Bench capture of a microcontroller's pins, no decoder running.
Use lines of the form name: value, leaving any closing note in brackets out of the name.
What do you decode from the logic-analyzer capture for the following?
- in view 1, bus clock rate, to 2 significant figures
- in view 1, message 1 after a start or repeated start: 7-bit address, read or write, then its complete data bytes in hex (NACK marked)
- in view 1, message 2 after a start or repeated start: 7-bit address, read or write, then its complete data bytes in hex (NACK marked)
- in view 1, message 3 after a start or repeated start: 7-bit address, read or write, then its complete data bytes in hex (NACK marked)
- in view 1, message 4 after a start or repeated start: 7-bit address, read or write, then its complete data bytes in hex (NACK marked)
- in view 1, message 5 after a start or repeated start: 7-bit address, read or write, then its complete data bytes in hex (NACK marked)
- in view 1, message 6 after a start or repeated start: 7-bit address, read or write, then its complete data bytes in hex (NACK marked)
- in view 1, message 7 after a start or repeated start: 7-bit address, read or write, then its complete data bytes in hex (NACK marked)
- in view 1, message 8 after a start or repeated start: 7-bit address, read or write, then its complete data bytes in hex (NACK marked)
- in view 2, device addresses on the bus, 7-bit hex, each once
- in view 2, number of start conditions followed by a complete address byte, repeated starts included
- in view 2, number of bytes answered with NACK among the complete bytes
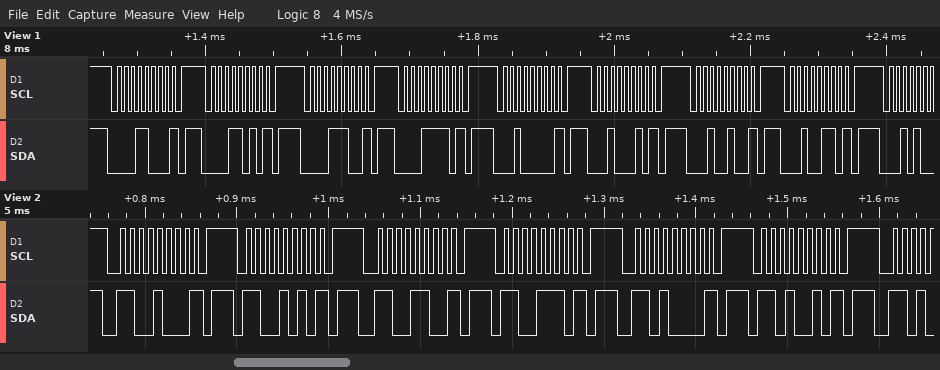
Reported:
in view 1, bus clock rate, to 2 significant figures: 100 kHz
in view 1, message 1 after a start or repeated start: 7-bit address, read or write, then its complete data bytes in hex: 0x0C write NACK
in view 1, message 2 after a start or repeated start: 7-bit address, read or write, then its complete data bytes in hex: 0x0D write NACK
in view 1, message 3 after a start or repeated start: 7-bit address, read or write, then its complete data bytes in hex: 0x0E write NACK
in view 1, message 4 after a start or repeated start: 7-bit address, read or write, then its complete data bytes in hex: 0x0F write NACK
in view 1, message 5 after a start or repeated start: 7-bit address, read or write, then its complete data bytes in hex: 0x10 write NACK
in view 1, message 6 after a start or repeated start: 7-bit address, read or write, then its complete data bytes in hex: 0x11 write NACK
in view 1, message 7 after a start or repeated start: 7-bit address, read or write, then its complete data bytes in hex: 0x12 write NACK
in view 1, message 8 after a start or repeated start: 7-bit address, read or write, then its complete data bytes in hex: 0x13 write NACK
in view 2, device addresses on the bus, 7-bit hex, each once: 0x64 0x65 0x66 0x67 0x68 0x69
in view 2, number of start conditions followed by a complete address byte, repeated starts included: 6
in view 2, number of bytes answered with NACK among the complete bytes: 6
